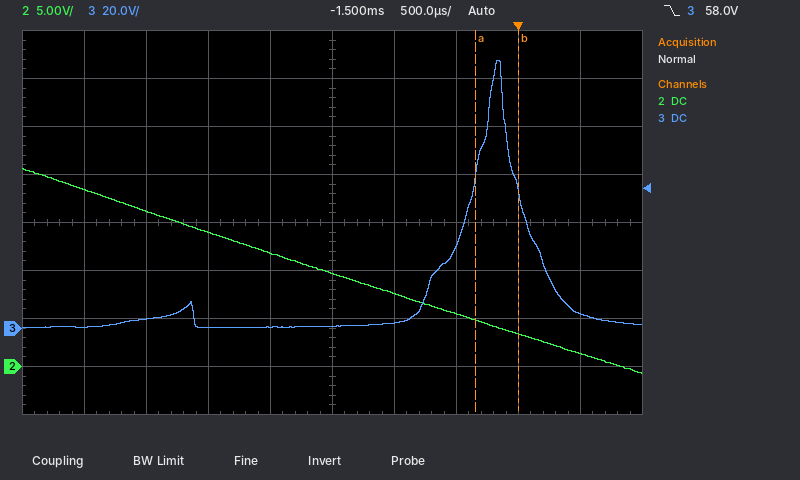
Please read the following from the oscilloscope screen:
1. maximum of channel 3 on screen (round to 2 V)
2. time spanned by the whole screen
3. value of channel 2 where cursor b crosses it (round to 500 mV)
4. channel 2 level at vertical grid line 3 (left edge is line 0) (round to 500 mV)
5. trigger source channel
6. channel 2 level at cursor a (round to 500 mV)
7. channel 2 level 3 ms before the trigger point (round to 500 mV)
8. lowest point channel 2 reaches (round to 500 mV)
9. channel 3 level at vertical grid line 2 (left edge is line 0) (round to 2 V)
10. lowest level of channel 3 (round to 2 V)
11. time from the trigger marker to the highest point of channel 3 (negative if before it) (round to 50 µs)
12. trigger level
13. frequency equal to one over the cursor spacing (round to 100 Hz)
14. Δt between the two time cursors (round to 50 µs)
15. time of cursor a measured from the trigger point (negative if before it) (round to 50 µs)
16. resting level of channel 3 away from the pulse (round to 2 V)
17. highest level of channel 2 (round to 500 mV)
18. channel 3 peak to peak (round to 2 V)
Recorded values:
112 V
5 ms
3.5 V
14.0 V
channel 3
5.0 V
16.0 V
-500 mV
4 V
0 V
-150 µs
58.0 V
2.9 kHz
350 µs
-350 µs
0 V
20.5 V
112 V
